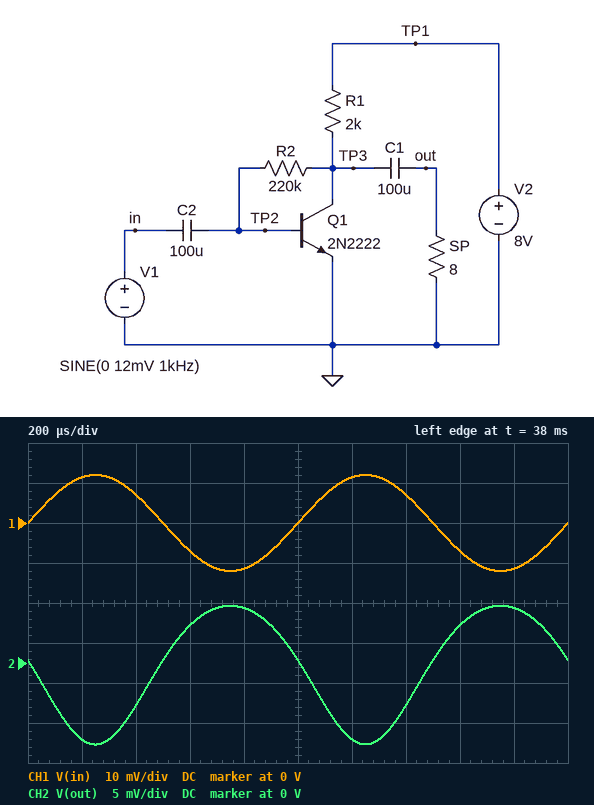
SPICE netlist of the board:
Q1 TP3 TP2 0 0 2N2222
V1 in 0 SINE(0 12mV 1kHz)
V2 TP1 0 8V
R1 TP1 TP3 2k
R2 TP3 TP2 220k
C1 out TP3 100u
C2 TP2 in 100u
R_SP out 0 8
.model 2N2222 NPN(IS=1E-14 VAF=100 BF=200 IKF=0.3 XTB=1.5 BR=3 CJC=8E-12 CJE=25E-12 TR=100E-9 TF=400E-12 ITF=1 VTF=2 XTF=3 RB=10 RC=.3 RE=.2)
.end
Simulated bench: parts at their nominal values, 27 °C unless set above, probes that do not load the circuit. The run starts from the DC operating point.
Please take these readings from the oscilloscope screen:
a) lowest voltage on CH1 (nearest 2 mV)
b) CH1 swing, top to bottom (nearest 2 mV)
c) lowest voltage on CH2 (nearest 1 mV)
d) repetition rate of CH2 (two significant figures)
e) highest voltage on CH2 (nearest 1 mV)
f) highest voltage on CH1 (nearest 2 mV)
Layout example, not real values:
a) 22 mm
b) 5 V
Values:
a) -12 mV
b) 24 mV
c) -10 mV
d) 1.0 kHz
e) 7 mV
f) 12 mV
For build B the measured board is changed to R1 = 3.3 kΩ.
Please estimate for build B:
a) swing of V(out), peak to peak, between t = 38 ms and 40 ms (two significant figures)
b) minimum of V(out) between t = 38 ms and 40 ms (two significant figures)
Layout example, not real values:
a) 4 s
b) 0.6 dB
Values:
a) 12 mV
b) -7.4 mV
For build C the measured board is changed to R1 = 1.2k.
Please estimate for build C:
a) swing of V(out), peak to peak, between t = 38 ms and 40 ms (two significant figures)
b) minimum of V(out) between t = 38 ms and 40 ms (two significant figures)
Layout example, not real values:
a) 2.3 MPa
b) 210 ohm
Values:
a) 23 mV
b) -13 mV
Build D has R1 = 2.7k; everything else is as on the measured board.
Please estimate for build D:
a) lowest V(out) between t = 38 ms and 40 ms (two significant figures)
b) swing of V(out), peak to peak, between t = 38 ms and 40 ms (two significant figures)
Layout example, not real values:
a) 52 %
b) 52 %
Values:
a) -8.4 mV
b) 14 mV
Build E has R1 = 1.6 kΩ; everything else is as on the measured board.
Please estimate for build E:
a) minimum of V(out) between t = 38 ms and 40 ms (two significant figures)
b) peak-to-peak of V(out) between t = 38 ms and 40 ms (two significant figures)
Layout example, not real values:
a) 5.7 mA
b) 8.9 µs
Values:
a) -12 mV
b) 20 mV
